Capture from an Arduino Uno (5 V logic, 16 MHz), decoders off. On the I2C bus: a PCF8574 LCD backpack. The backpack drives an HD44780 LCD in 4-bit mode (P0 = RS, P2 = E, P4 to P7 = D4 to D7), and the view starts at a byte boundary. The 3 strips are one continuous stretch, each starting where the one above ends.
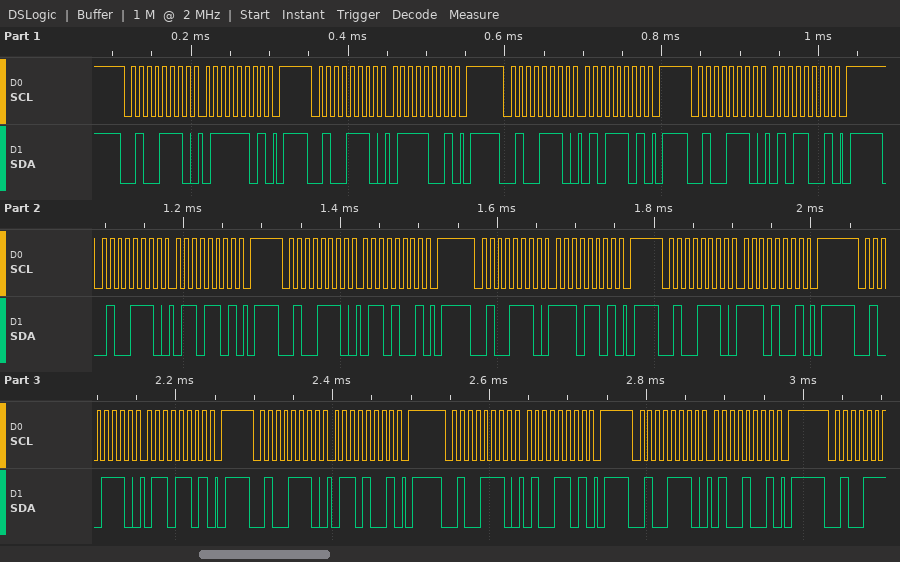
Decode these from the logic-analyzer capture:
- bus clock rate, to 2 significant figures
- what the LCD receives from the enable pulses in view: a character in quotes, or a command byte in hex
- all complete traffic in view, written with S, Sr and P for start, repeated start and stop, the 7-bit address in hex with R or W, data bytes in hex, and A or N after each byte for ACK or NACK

100 kHz
'u' 'n' 'd'
S 27W A 7D A P S 27W A 79 A P S 27W A 5D A P S 27W A 59 A P S 27W A 6D A P S 27W A 69 A P S 27W A ED A P S 27W A E9 A P S 27W A 6D A P S 27W A 69 A P S 27W A 4D A P S 27W A 49 A P
